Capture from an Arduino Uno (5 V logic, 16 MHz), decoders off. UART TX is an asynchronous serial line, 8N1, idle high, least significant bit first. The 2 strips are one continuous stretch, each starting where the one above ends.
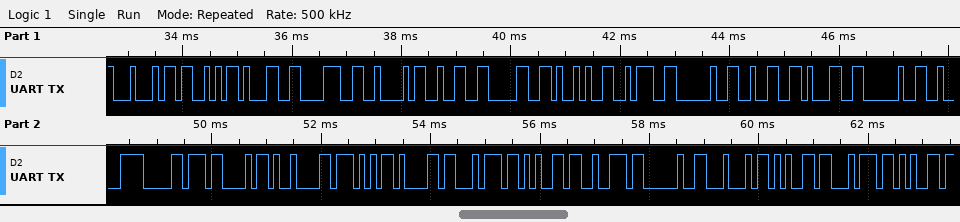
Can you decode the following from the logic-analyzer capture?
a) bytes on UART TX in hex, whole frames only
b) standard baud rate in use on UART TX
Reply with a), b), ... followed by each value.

a) 44 53 31 38 42 32 30 29 3A 20 32 31 20 C2 B0 43 09 57 61 74 65 72 20 44 65 74 65
b) 9600 baud
